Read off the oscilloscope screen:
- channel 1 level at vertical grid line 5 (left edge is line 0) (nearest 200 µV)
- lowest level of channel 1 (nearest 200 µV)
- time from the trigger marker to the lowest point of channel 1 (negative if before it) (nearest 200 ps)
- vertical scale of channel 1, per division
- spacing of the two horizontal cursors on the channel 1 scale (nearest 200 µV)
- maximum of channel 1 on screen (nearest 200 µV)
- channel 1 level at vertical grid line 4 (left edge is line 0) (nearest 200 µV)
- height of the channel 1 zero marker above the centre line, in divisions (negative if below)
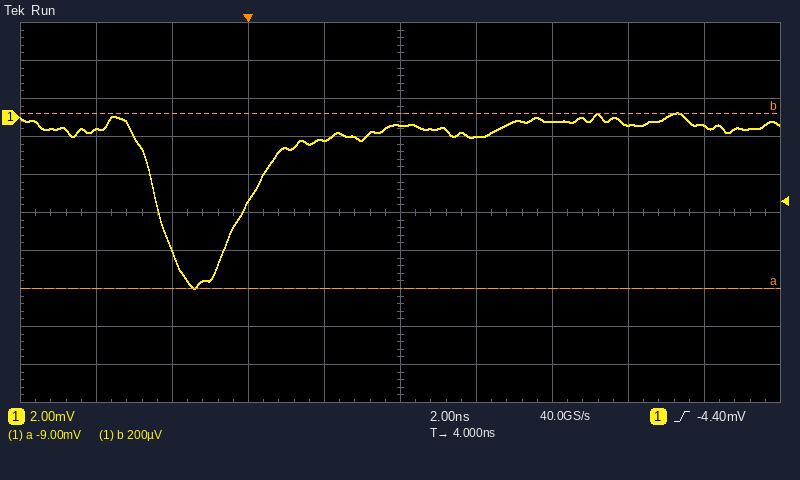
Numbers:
-400 µV
-9.0 mV
-1.4 ns
2 mV
9.2 mV
200 µV
-1.2 mV
+2.5 div
